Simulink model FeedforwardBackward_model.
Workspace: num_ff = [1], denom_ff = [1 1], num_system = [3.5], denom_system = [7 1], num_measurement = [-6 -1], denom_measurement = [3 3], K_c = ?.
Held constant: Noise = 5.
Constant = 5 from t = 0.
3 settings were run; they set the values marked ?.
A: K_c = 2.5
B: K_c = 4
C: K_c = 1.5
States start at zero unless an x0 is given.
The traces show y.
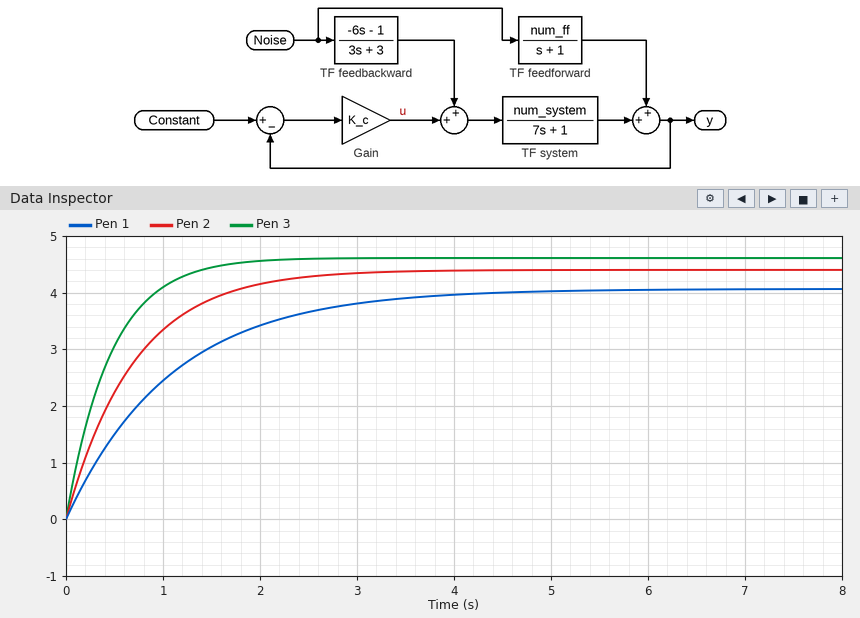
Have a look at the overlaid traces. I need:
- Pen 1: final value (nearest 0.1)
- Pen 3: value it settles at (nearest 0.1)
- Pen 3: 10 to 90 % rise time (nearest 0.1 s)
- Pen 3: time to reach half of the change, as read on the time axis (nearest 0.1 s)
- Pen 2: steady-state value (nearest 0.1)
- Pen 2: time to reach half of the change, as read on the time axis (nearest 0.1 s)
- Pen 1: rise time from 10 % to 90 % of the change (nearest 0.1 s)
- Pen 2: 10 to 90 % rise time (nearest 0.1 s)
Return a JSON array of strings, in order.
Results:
["4.1", "4.6", "1.0 s", "0.3 s", "4.4", "0.5 s", "2.4 s", "1.5 s"]
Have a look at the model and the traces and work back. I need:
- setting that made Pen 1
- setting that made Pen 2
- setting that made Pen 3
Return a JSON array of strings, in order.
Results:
["C", "A", "B"]
